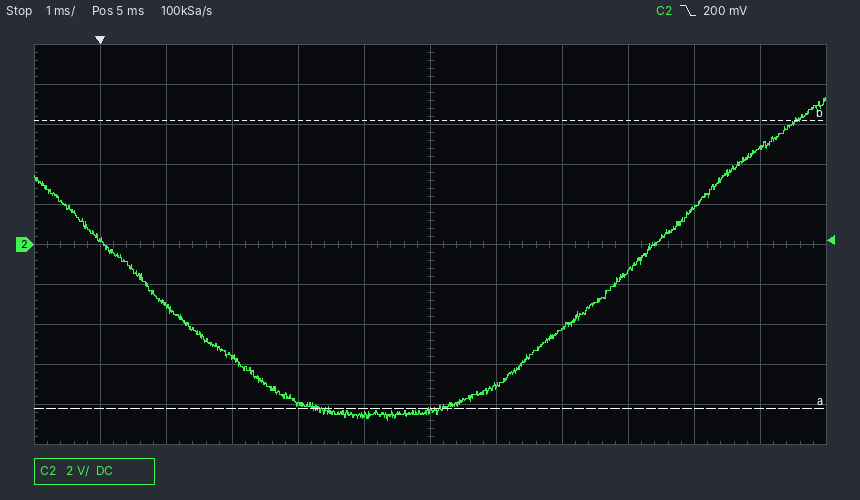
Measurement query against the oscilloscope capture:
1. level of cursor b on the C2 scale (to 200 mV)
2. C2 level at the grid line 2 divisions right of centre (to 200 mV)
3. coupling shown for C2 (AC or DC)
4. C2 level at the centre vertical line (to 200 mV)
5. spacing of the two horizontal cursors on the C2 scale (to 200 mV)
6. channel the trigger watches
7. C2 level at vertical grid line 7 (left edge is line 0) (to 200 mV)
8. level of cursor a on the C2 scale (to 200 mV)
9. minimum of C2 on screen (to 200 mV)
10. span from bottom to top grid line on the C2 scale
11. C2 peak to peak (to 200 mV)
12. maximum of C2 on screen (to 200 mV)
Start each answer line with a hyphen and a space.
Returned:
- 6.2 V
- -4.2 V
- DC
- -8.4 V
- 14.4 V
- C2
- -7.0 V
- -8.2 V
- -8.8 V
- 20 V
- 16.2 V
- 7.4 V
